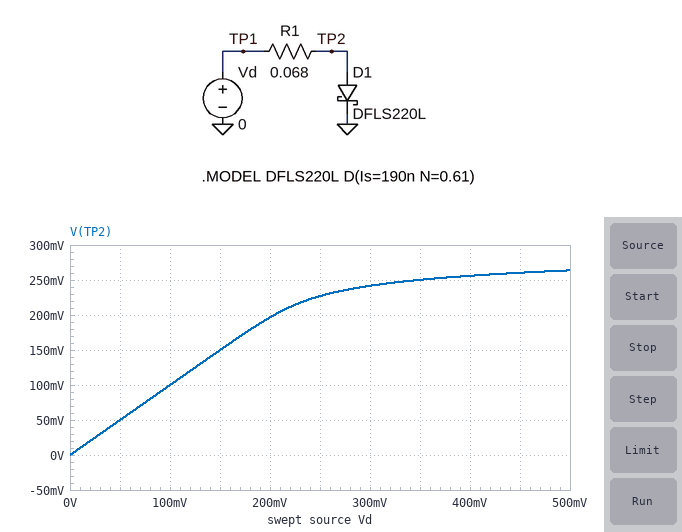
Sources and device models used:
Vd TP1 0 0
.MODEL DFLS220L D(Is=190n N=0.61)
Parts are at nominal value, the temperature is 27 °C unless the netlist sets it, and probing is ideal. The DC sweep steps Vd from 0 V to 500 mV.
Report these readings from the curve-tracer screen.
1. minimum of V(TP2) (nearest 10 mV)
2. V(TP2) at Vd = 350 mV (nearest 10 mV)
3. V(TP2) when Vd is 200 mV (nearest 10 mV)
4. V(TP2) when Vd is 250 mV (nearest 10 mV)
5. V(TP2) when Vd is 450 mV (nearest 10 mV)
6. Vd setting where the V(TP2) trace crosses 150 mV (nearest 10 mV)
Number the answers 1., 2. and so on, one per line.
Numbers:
1. 0 V
2. 250 mV
3. 200 mV
4. 230 mV
5. 260 mV
6. 150 mV
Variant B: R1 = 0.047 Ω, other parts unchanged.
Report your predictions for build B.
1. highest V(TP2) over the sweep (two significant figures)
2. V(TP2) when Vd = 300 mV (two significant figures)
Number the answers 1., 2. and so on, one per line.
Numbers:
1. 270 mV
2. 250 mV
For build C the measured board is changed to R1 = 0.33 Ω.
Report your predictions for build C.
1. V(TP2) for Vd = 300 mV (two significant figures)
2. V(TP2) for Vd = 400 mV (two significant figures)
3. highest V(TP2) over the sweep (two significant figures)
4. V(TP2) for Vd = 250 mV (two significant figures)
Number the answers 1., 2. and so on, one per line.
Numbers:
1. 220 mV
2. 230 mV
3. 240 mV
4. 210 mV
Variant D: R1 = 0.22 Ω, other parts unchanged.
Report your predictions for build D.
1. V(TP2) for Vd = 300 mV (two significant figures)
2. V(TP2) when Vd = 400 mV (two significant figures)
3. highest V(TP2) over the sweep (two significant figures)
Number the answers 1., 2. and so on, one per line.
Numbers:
1. 230 mV
2. 240 mV
3. 250 mV
